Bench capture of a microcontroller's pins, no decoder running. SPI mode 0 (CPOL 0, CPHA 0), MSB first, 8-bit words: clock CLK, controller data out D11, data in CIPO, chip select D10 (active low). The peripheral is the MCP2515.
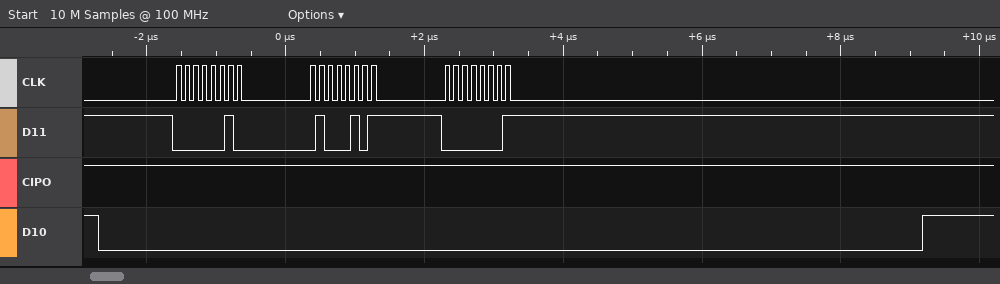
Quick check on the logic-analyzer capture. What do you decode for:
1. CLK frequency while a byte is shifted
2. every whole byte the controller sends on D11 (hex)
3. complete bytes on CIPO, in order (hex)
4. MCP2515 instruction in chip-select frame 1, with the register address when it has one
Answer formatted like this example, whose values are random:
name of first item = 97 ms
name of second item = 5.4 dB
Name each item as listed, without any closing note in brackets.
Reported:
CLK frequency while a byte is shifted = 8 MHz
every whole byte the controller sends on D11 = 02 45 01
complete bytes on CIPO, in order = FF FF FF
MCP2515 instruction in chip-select frame 1, with the register address when it has one = WRITE 0x45
